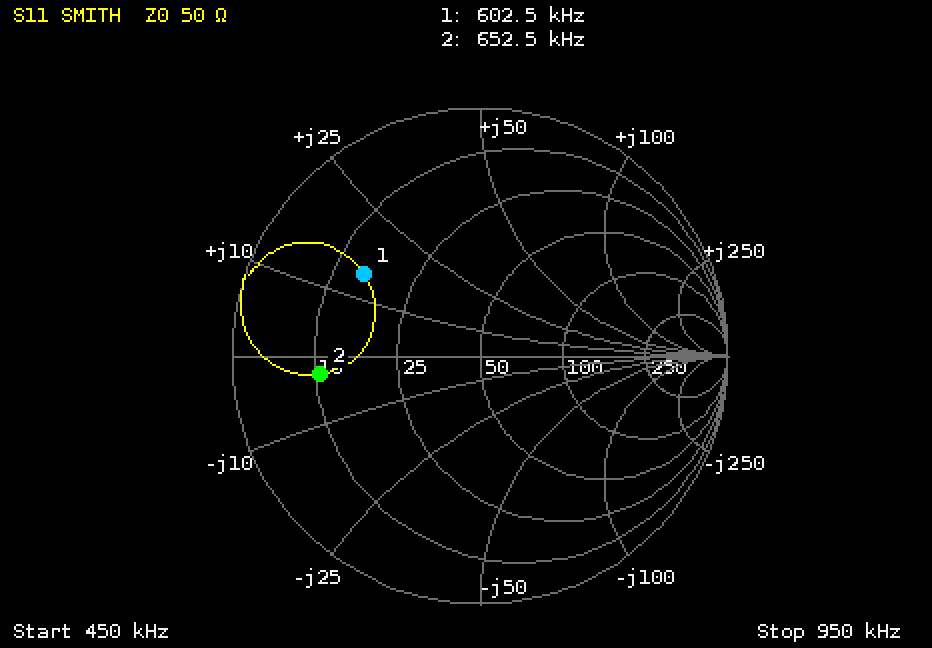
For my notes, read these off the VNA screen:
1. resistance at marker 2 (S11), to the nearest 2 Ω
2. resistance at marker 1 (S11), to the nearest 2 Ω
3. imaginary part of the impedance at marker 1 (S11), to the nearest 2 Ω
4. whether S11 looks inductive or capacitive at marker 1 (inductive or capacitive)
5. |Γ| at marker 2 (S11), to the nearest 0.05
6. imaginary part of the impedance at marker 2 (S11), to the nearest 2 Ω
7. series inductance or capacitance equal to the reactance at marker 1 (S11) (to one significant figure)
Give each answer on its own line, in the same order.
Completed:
10 Ω
14 Ω
+14 Ω
inductive
0.65
-2 Ω
4 µH
